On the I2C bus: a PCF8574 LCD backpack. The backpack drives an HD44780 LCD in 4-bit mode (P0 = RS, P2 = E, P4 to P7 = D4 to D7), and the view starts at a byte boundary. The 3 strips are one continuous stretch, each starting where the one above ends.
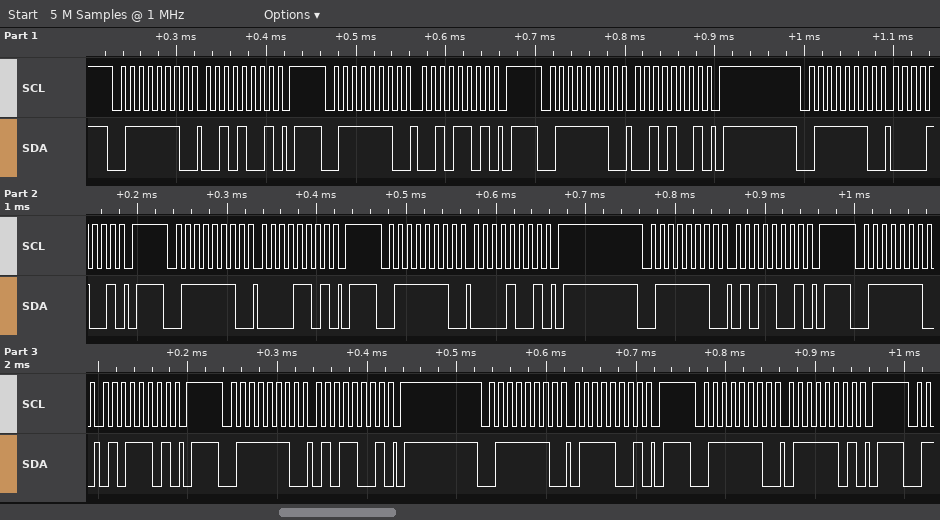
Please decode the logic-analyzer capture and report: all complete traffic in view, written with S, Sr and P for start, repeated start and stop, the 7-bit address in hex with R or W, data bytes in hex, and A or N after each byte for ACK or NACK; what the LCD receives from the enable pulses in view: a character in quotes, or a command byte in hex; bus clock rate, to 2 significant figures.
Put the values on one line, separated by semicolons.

S 3FW A 29 A P S 3FW A 2D A P S 3FW A 29 A P S 3FW A 09 A P S 3FW A 0D A P S 3FW A 09 A P S 3FW A 59 A P S 3FW A 5D A P S 3FW A 59 A P S 3FW A 79 A P S 3FW A 7D A P; ' '; 100 kHz
